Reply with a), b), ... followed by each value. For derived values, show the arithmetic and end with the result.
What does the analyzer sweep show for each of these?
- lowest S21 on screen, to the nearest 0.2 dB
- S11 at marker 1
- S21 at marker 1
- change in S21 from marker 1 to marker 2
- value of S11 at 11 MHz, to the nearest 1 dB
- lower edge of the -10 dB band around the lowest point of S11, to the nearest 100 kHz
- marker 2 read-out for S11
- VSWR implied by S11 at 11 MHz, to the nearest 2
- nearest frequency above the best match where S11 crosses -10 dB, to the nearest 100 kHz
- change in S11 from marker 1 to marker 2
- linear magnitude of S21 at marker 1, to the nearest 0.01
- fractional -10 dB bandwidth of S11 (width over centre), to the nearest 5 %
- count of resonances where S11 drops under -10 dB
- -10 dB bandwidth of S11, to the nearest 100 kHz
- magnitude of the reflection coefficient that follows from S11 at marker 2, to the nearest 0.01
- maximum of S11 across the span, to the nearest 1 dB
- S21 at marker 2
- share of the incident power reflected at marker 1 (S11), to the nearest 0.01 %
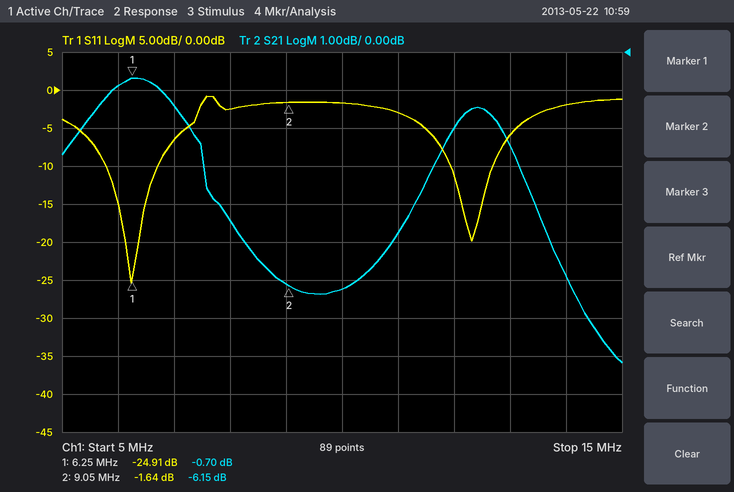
a) -8.2 dB
b) -24.91 dB
c) -0.70 dB
d) -6.15 − (-0.7) = -5.45 dB
e) -3 dB
f) 5.8 MHz
g) -1.64 dB
h) |Γ| = 10^(-3/20) = 0.7079; VSWR = (1 + 0.7079)/(1 − 0.7079) ≈ 6
i) 6.7 MHz
j) -1.64 − (-24.91) = 23.27 dB
k) 10^(-0.7/20) ≈ 0.92
l) 900 kHz / 6.25 MHz ≈ 14.4 %, so 15 % to the nearest 5 %
m) 2
n) 6.7 MHz − 5.8 MHz = 900 kHz
o) 10^(-1.64/20) ≈ 0.83
p) -1 dB
q) -6.15 dB
r) 10^(-24.91/10) ≈ 0.32 %
